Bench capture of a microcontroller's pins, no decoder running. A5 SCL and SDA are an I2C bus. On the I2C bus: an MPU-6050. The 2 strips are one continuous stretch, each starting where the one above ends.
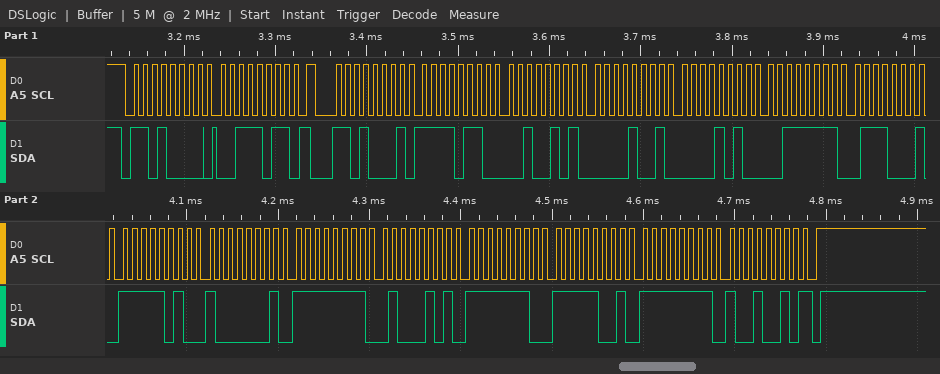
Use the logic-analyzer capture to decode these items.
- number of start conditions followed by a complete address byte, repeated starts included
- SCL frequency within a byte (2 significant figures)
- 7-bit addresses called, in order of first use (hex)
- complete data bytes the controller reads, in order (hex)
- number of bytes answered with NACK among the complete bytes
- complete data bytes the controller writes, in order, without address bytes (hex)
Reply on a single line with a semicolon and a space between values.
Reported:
2; 100 kHz; 0x68; F6 25 09 0A 3F 71 FA 81 FF 45 FE F9 FF 92; 1; 3B
